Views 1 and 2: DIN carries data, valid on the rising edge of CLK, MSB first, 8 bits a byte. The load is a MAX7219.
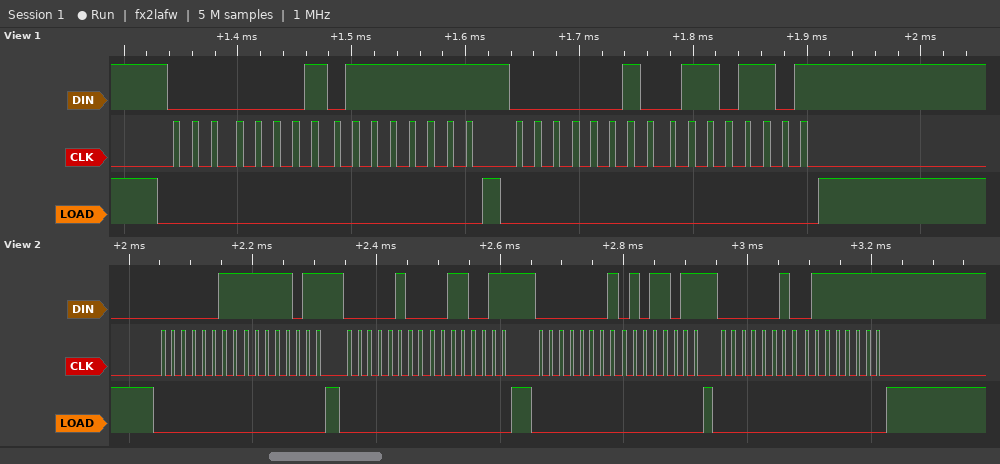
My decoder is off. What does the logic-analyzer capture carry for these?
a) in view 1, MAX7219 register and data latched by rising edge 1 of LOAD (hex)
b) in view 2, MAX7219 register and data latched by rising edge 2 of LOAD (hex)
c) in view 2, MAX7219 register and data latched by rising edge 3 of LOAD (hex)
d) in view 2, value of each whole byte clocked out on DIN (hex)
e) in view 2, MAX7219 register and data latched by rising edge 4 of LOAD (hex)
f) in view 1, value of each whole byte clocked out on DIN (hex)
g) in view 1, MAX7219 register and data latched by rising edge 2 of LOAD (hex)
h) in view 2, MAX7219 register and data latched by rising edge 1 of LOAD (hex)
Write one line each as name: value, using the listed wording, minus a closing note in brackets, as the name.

in view 1, MAX7219 register and data latched by rising edge 1 of LOAD: register 0x1, data 0x7F
in view 2, MAX7219 register and data latched by rising edge 2 of LOAD: register 0x4, data 0x33
in view 2, MAX7219 register and data latched by rising edge 3 of LOAD: register 0x1, data 0x5B
in view 2, value of each whole byte clocked out on DIN: 03 FB 04 33 01 5B 02 7F
in view 2, MAX7219 register and data latched by rising edge 4 of LOAD: register 0x2, data 0x7F
in view 1, value of each whole byte clocked out on DIN: 0x01 0x7F 0x02 0x6D
in view 1, MAX7219 register and data latched by rising edge 2 of LOAD: register 0x2, data 0x6D
in view 2, MAX7219 register and data latched by rising edge 1 of LOAD: register 0x3, data 0xFB
